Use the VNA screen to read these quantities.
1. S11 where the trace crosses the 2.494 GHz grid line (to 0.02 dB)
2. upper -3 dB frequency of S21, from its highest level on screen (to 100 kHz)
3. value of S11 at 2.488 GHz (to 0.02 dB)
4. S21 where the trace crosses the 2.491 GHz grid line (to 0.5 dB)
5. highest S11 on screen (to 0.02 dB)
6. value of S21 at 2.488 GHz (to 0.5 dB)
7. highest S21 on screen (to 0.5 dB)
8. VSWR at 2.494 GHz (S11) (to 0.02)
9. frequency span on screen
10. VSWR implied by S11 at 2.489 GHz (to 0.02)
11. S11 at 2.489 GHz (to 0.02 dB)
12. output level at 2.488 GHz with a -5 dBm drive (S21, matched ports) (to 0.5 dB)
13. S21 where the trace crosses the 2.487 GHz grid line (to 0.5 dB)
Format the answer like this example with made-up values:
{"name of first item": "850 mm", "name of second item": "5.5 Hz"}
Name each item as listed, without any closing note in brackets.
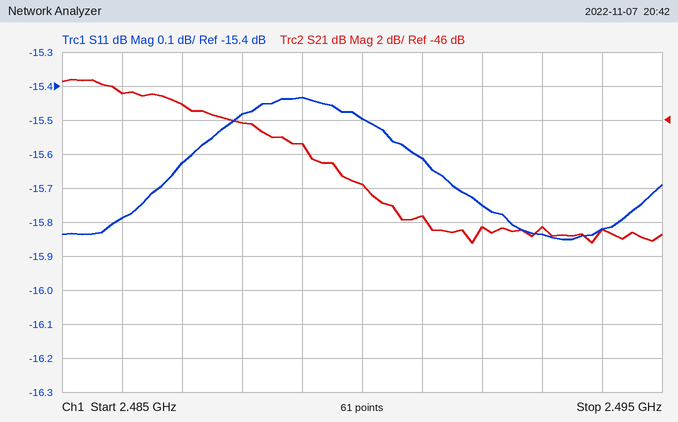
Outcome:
{"S11 where the trace crosses the 2.494 GHz grid line": "-15.82 dB", "upper -3 dB frequency of S21, from its highest level on screen": "2.4883 GHz", "value of S11 at 2.488 GHz": "-15.48 dB", "S21 where the trace crosses the 2.491 GHz grid line": "-51.5 dB", "highest S11 on screen": "-15.44 dB", "value of S21 at 2.488 GHz": "-46.0 dB", "highest S21 on screen": "-43.5 dB", "VSWR at 2.494 GHz (S11)": "1.38", "frequency span on screen": "10 MHz", "VSWR implied by S11 at 2.489 GHz": "1.40", "S11 at 2.489 GHz": "-15.44 dB", "output level at 2.488 GHz with a -5 dBm drive (S21, matched ports)": "-51.0 dBm", "S21 where the trace crosses the 2.487 GHz grid line": "-45.0 dB"}
